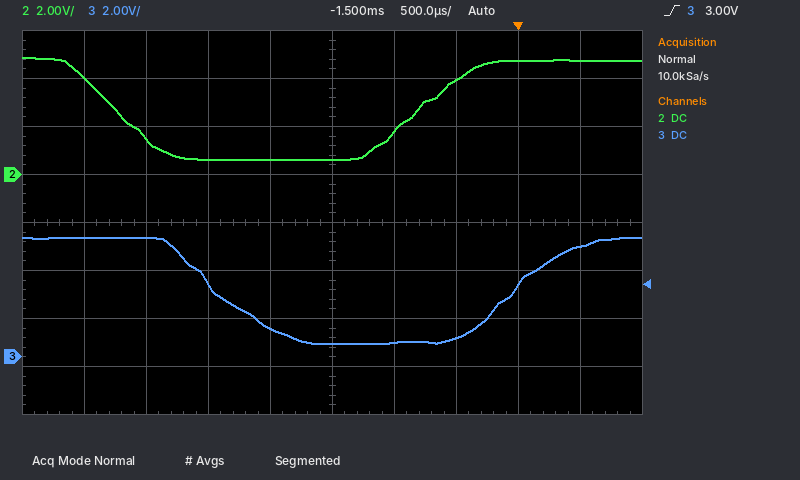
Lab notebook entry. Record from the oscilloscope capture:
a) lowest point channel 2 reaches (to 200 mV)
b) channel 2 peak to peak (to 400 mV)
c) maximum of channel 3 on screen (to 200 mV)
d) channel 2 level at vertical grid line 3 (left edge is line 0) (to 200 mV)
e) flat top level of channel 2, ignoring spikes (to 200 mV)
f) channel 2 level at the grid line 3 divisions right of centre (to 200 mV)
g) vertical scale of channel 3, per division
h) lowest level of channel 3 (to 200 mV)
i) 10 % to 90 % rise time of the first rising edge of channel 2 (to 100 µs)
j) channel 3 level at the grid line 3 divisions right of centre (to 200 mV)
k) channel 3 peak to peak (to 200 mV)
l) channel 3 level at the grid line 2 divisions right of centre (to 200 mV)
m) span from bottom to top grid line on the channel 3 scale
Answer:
600 mV
4.4 V
5.0 V
600 mV
4.8 V
4.8 V
2 V
600 mV
800 µs
3.0 V
4.4 V
800 mV
16 V
